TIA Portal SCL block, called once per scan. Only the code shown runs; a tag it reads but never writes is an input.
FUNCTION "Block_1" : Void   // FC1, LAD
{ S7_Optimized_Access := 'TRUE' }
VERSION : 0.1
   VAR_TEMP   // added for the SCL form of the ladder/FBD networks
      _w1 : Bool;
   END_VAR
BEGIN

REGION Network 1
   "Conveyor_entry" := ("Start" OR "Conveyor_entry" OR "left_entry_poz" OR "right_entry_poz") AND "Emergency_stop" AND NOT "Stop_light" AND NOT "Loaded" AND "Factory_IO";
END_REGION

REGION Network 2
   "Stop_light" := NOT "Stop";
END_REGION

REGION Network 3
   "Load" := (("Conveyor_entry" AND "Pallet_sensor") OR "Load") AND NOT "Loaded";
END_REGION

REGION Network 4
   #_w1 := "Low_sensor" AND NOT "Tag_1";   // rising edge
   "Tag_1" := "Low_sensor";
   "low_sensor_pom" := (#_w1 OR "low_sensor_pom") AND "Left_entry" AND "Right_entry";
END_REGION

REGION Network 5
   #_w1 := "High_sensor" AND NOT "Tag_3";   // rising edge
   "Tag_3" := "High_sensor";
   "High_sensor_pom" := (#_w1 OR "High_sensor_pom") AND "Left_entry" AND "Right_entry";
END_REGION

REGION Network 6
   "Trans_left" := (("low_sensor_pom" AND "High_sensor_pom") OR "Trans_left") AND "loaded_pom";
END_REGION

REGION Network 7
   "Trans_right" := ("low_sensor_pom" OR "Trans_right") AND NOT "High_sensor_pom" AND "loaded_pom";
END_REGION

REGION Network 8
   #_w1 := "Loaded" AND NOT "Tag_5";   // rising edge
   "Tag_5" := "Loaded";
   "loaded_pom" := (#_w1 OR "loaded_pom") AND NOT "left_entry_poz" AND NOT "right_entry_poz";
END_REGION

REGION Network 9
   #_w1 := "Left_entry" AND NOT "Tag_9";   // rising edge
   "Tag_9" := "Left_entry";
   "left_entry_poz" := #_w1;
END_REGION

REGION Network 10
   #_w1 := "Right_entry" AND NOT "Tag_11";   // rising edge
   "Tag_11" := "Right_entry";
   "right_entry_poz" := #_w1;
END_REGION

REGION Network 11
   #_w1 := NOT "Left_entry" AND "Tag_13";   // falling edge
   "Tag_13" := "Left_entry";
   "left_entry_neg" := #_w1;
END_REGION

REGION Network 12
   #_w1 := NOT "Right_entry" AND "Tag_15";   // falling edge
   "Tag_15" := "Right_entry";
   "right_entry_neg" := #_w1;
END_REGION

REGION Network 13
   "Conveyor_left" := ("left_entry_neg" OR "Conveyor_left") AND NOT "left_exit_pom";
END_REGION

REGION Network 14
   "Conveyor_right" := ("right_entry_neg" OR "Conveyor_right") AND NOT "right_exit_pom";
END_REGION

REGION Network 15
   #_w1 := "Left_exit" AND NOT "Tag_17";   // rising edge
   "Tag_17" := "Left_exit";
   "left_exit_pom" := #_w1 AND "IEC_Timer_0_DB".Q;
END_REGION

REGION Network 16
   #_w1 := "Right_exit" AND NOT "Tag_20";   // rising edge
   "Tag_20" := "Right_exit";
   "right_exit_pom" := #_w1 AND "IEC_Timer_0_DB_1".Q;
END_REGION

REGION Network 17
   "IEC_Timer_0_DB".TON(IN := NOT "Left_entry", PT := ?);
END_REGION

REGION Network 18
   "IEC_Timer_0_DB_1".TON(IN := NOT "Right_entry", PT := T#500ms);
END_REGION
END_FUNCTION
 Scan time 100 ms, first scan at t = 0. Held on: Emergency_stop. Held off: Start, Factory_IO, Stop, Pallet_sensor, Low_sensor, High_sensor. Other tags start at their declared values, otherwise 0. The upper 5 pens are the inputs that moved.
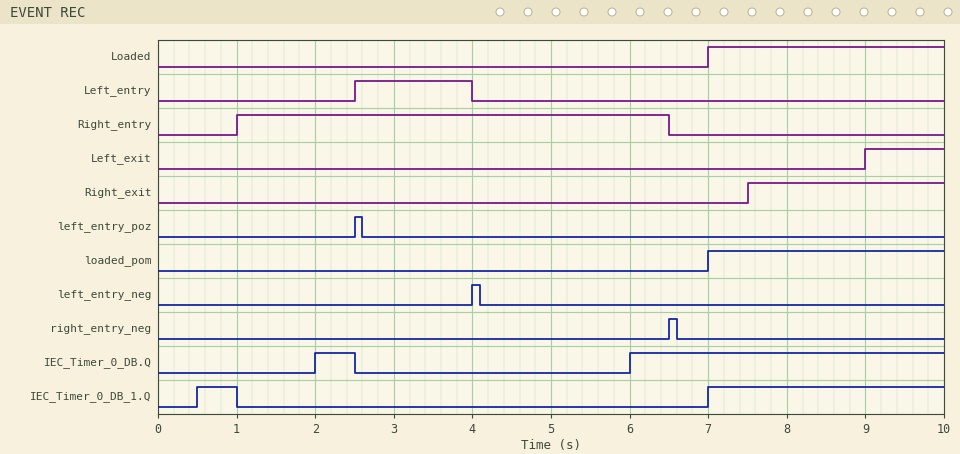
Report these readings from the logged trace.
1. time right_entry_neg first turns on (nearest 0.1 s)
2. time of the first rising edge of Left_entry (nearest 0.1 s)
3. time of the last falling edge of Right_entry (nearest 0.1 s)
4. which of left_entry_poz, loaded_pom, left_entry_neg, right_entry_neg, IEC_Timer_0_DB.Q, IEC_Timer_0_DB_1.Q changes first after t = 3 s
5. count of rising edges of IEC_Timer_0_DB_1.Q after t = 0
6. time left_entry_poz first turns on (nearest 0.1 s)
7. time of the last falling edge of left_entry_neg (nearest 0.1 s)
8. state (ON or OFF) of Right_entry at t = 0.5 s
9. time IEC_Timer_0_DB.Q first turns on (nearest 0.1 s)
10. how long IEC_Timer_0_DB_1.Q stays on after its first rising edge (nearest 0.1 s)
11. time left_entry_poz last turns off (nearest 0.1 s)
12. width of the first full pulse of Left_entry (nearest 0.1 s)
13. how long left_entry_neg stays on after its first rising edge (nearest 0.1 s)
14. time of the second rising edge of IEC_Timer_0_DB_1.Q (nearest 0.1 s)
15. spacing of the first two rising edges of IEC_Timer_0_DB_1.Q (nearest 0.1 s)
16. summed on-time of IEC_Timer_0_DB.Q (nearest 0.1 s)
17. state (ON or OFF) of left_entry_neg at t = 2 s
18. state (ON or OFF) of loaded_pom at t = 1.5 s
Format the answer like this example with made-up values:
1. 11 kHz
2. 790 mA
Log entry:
1. 6.5 s
2. 2.5 s
3. 6.5 s
4. left_entry_neg
5. 2
6. 2.5 s
7. 4.1 s
8. OFF
9. 2.0 s
10. 0.5 s
11. 2.6 s
12. 1.5 s
13. 0.1 s
14. 7.0 s
15. 6.5 s
16. 4.5 s
17. OFF
18. OFF
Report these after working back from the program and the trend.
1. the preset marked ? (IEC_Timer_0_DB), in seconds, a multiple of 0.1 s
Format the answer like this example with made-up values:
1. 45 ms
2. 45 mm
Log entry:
1. 2.0 s
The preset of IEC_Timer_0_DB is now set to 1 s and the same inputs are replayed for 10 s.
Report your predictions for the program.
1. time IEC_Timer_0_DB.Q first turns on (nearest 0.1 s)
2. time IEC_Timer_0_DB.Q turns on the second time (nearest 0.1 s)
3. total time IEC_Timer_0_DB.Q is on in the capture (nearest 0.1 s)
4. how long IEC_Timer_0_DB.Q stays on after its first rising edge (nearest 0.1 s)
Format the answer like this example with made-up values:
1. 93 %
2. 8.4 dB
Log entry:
1. 1.0 s
2. 5.0 s
3. 6.5 s
4. 1.5 s
